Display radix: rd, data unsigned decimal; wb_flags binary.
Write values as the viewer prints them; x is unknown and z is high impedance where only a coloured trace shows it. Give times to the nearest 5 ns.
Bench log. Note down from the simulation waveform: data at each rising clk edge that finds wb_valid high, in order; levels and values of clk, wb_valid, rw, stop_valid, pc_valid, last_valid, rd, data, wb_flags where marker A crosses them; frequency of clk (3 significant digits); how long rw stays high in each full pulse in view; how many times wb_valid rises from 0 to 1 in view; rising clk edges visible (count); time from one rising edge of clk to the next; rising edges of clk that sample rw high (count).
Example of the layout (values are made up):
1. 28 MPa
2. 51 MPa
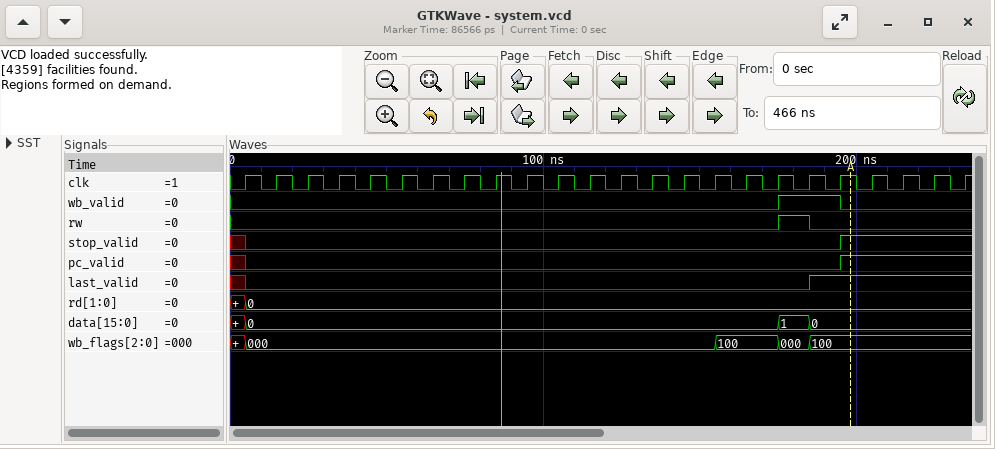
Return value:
1. 1, 0
2. clk=1, wb_valid=0, rw=0, stop_valid=1, pc_valid=1, last_valid=1, rd=0, data=0, wb_flags=100
3. 100 MHz
4. 10 ns
5. 1
6. 24
7. 10 ns
8. 1
